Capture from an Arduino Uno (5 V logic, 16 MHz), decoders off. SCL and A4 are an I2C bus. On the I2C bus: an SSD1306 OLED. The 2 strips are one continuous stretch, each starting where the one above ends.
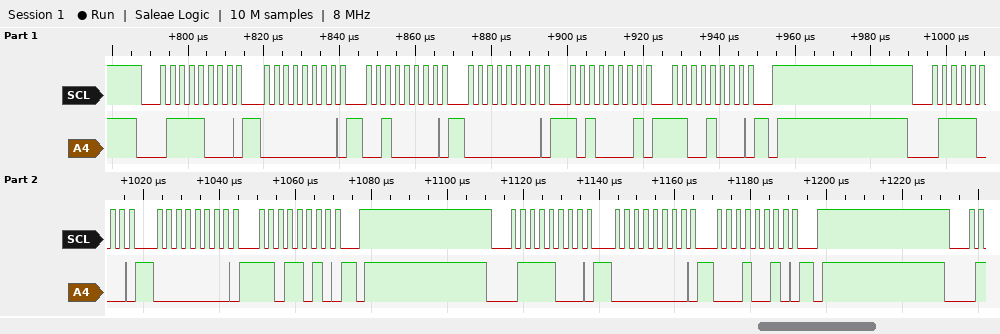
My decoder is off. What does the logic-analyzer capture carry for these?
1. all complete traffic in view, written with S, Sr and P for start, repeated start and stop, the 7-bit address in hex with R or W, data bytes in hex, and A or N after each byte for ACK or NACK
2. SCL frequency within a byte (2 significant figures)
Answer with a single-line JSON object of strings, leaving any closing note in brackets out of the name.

{"all complete traffic in view, written with S, Sr and P for start, repeated start and stop, the 7-bit address in hex with R or W, data bytes in hex, and A or N after each byte for ACK or NACK": "S 3CW A 00 A 20 A 00 A A1 A C8 A P S 3CW A 00 A DA A P S 3CW A 00 A 12 A P", "SCL frequency within a byte": "400 kHz"}
